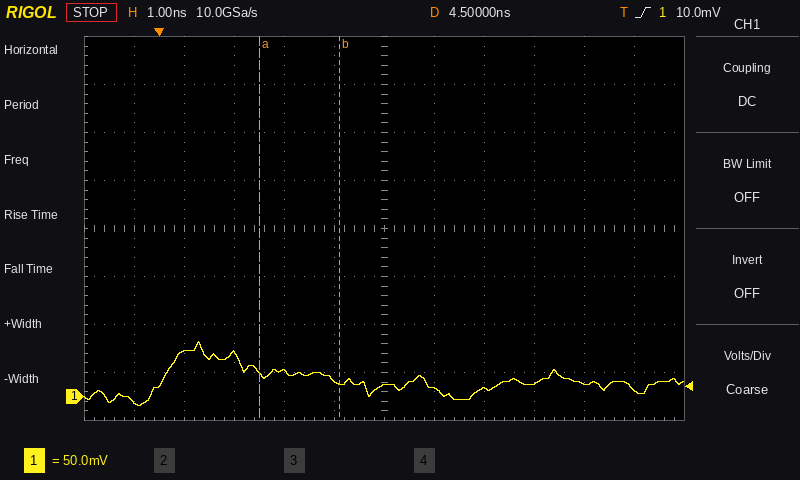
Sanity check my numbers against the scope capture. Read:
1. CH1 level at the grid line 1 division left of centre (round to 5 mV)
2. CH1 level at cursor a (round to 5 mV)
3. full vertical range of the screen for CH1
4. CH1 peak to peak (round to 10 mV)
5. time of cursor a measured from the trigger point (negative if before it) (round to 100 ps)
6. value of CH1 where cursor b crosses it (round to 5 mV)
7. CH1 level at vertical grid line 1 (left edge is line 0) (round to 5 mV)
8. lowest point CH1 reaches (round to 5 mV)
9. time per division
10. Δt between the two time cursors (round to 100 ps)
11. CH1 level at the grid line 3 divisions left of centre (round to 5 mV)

15 mV
25 mV
400 mV
70 mV
+2.0 ns
15 mV
-5 mV
-10 mV
1 ns
1.6 ns
45 mV
